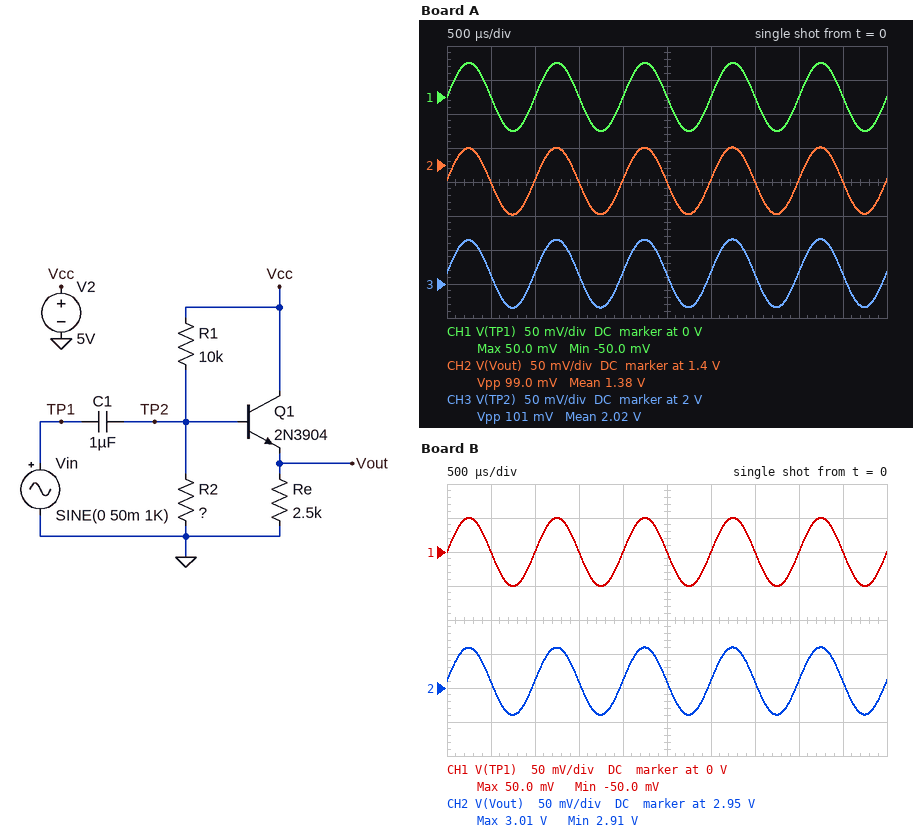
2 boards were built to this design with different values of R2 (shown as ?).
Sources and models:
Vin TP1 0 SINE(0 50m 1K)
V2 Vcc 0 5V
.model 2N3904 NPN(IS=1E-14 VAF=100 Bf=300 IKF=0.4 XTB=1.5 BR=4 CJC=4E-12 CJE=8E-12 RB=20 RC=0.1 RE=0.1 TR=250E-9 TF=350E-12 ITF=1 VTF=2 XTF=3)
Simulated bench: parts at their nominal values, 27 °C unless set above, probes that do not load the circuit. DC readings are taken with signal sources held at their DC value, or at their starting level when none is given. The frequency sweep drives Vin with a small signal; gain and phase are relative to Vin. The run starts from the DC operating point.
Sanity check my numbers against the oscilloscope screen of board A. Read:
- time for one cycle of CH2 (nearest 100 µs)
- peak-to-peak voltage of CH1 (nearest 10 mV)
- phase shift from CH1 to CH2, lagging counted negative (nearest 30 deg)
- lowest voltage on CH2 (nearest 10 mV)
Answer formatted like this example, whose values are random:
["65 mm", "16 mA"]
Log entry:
["1.0 ms", "100 mV", "0 deg", "1.33 V"]
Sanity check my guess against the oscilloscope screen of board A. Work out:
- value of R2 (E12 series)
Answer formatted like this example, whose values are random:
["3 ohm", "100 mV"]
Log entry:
["6.8 kΩ"]
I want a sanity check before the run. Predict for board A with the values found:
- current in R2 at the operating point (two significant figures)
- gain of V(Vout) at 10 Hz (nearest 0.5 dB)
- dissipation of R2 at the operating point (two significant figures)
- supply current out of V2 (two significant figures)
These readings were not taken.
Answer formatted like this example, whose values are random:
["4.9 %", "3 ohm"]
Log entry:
["300 µA", "-12.5 dB", "600 µW", "850 µA"]
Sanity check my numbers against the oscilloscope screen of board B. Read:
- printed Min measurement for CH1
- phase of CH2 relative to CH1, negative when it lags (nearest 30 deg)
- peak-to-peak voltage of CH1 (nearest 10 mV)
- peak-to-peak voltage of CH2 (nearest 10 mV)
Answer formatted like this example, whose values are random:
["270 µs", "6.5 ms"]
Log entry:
["-50.0 mV", "0 deg", "100 mV", "100 mV"]
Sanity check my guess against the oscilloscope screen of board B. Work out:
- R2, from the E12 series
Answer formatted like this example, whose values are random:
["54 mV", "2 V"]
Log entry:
["27 kΩ"]
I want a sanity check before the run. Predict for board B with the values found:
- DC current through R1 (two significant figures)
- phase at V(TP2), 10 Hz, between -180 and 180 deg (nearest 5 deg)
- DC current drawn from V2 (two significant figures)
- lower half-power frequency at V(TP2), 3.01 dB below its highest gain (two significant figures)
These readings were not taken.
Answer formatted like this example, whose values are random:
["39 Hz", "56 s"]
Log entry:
["140 µA", "65 deg", "1.3 mA", "22 Hz"]
